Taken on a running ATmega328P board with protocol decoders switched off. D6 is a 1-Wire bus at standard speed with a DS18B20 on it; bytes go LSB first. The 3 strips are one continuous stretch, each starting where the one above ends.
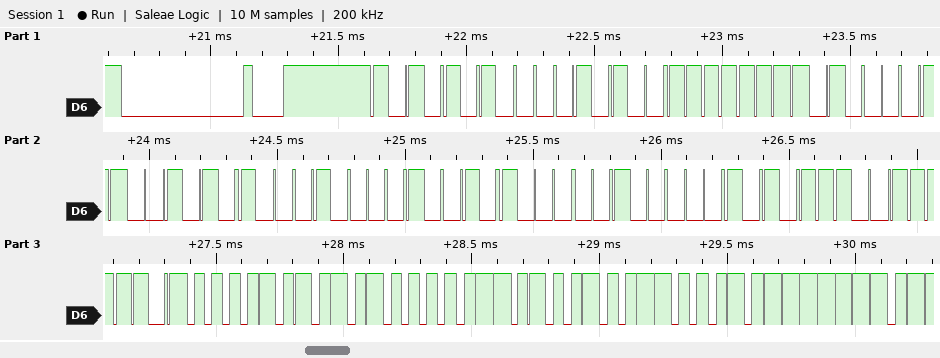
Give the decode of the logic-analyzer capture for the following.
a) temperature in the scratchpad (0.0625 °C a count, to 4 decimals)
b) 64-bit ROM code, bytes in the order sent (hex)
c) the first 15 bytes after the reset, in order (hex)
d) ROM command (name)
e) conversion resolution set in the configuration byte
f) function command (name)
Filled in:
85.0000 °C
28 FF C2 54 84 14 04 75
55 28 FF C2 54 84 14 04 75 BE 50 05 4B 46 7F
Match ROM
12 bits
Read Scratchpad
